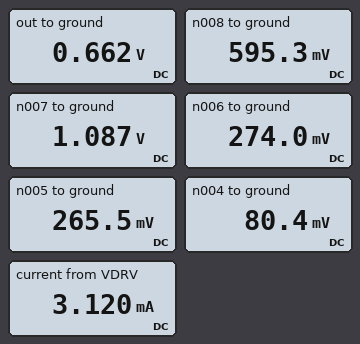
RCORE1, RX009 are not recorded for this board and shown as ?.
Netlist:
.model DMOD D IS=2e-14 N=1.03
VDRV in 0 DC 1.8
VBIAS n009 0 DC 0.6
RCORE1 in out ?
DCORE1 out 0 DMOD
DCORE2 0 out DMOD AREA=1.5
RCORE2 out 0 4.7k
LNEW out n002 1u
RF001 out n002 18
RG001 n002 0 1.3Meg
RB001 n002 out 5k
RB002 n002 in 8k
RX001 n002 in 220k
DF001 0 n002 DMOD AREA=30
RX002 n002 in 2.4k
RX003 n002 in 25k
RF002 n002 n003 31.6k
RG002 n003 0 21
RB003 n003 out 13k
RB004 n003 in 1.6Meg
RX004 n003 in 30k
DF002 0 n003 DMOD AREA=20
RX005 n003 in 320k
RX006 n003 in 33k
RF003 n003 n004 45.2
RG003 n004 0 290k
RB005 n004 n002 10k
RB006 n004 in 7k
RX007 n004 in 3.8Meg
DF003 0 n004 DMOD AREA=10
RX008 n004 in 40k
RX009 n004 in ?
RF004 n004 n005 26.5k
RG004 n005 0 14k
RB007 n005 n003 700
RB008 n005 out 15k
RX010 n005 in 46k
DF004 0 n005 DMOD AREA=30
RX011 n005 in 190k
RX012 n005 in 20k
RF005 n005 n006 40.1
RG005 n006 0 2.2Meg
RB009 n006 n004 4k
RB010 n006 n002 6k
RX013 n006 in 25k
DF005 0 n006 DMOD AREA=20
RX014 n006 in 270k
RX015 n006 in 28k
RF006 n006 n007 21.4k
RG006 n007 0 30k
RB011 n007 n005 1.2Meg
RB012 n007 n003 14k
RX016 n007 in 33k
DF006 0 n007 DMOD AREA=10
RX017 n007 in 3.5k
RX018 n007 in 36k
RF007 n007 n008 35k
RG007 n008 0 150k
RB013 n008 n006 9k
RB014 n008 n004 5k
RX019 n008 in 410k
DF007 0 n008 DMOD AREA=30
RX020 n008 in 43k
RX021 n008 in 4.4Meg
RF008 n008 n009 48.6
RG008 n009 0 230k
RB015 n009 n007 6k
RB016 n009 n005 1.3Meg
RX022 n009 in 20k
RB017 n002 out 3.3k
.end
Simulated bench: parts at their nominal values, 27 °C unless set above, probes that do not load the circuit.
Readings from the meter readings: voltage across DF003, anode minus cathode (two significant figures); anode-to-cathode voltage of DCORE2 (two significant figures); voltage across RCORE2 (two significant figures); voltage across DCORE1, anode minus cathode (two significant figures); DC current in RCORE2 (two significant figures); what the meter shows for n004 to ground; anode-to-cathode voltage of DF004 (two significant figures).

-80 mV
-660 mV
660 mV
660 mV
140 µA
80.4 mV
-270 mV
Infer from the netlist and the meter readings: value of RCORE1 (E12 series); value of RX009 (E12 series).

1.2 kΩ
3.3 kΩ
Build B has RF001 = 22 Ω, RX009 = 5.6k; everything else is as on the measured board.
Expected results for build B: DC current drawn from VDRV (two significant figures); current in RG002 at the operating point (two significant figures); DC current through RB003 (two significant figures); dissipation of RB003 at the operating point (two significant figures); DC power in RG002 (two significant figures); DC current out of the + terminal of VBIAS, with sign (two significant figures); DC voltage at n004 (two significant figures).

2.9 mA
1.4 mA
49 µA
31 µW
42 µW
-38 µA
67 mV
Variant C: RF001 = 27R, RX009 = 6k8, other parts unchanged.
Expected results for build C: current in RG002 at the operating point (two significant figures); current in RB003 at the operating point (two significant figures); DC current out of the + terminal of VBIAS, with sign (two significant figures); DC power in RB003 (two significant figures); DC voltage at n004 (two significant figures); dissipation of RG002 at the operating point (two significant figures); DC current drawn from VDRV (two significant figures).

1.4 mA
49 µA
-37 µA
31 µW
64 mV
39 µW
2.9 mA
